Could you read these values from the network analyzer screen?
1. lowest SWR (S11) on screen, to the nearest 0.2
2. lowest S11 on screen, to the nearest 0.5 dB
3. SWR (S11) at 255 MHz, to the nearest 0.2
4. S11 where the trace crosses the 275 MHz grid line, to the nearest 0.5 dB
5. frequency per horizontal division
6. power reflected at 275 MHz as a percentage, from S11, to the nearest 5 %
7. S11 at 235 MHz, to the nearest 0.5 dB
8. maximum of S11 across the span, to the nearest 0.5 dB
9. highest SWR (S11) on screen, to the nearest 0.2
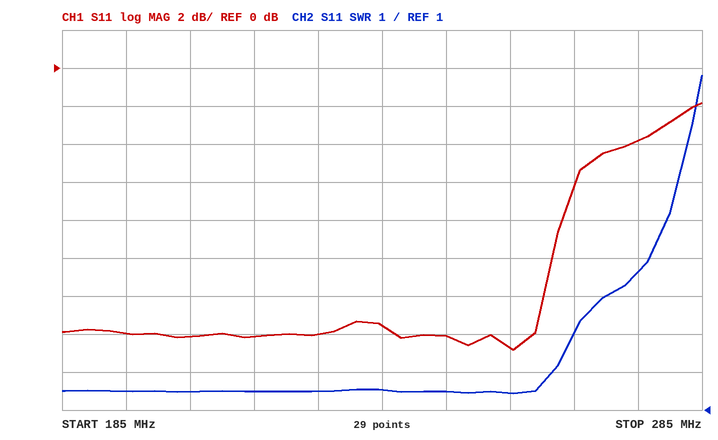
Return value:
1.4
-15.0 dB
1.4
-4.0 dB
10 MHz
40 %
-13.5 dB
-2.0 dB
9.8
